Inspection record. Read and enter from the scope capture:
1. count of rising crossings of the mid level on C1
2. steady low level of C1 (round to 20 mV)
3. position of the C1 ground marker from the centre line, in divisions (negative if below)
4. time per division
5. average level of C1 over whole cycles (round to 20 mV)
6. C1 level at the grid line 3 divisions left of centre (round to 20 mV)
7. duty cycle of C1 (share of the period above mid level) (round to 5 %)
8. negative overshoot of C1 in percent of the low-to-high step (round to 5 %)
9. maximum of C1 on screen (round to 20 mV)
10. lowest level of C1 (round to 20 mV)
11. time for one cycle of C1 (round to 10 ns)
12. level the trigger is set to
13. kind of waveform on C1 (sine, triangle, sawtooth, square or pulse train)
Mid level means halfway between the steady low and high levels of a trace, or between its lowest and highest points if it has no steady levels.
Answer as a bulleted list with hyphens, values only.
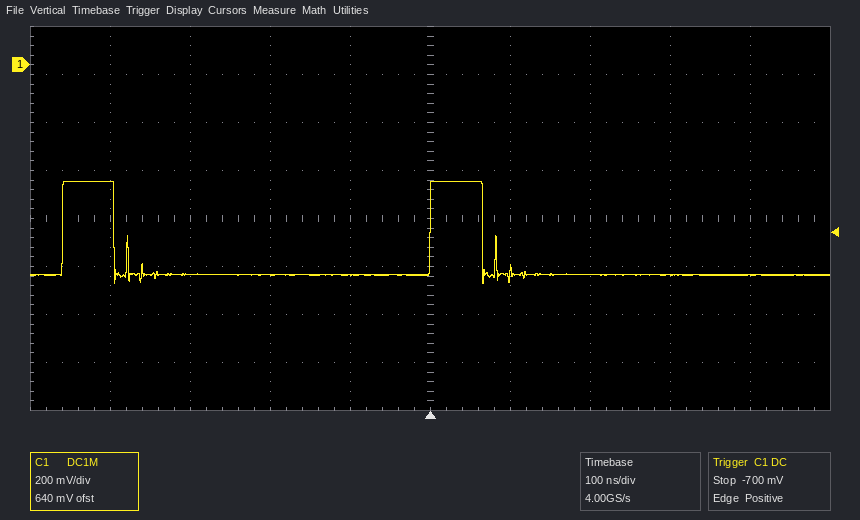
- 2
- -880 mV
- +3.2 div
- 100 ns
- -820 mV
- -880 mV
- 15 %
- 10 %
- -480 mV
- -920 mV
- 460 ns
- -700 mV
- pulse train
